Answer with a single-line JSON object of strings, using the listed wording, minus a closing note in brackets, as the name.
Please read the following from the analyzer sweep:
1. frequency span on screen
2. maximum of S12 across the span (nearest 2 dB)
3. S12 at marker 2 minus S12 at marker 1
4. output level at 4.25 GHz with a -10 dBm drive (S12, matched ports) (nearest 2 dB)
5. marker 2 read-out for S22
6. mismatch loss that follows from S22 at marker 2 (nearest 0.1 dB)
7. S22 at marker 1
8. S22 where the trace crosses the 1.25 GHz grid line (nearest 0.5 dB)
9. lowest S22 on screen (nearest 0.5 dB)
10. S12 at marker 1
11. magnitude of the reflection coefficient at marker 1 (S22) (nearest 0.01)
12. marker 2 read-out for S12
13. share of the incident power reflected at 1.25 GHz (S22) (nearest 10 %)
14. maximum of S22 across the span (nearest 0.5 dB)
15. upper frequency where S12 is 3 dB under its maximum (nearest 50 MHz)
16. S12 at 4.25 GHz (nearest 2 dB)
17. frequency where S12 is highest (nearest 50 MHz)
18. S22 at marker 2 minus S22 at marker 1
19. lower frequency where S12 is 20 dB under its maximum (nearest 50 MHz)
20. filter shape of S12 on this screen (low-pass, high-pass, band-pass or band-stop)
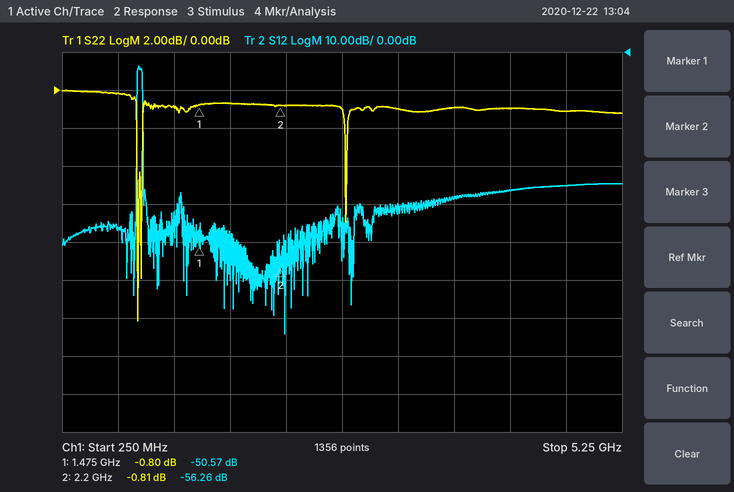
{"frequency span on screen": "5 GHz", "maximum of S12 across the span": "-4 dB", "S12 at marker 2 minus S12 at marker 1": "-5.69 dB", "output level at 4.25 GHz with a -10 dBm drive (S12, matched ports)": "-46 dBm", "marker 2 read-out for S22": "-0.81 dB", "mismatch loss that follows from S22 at marker 2": "7.7 dB", "S22 at marker 1": "-0.80 dB", "S22 where the trace crosses the 1.25 GHz grid line": "-1.0 dB", "lowest S22 on screen": "-12.0 dB", "S12 at marker 1": "-50.57 dB", "magnitude of the reflection coefficient at marker 1 (S22)": "0.91", "marker 2 read-out for S12": "-56.26 dB", "share of the incident power reflected at 1.25 GHz (S22)": "80 %", "maximum of S22 across the span": "0.0 dB", "upper frequency where S12 is 3 dB under its maximum": "950 MHz", "S12 at 4.25 GHz": "-36 dB", "frequency where S12 is highest": "950 MHz", "S22 at marker 2 minus S22 at marker 1": "-0.01 dB", "lower frequency where S12 is 20 dB under its maximum": "900 MHz", "filter shape of S12 on this screen": "band-pass"}
